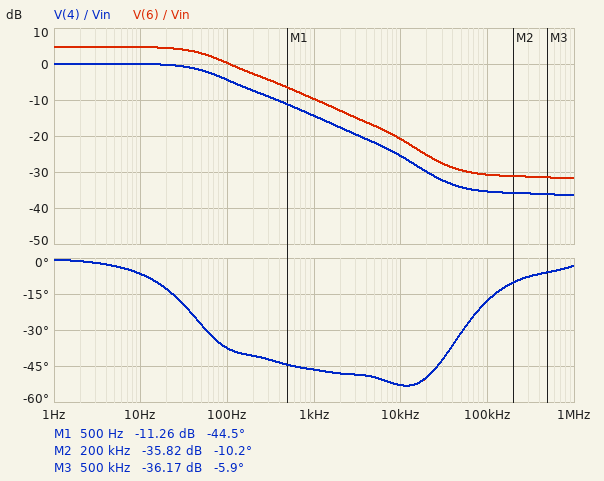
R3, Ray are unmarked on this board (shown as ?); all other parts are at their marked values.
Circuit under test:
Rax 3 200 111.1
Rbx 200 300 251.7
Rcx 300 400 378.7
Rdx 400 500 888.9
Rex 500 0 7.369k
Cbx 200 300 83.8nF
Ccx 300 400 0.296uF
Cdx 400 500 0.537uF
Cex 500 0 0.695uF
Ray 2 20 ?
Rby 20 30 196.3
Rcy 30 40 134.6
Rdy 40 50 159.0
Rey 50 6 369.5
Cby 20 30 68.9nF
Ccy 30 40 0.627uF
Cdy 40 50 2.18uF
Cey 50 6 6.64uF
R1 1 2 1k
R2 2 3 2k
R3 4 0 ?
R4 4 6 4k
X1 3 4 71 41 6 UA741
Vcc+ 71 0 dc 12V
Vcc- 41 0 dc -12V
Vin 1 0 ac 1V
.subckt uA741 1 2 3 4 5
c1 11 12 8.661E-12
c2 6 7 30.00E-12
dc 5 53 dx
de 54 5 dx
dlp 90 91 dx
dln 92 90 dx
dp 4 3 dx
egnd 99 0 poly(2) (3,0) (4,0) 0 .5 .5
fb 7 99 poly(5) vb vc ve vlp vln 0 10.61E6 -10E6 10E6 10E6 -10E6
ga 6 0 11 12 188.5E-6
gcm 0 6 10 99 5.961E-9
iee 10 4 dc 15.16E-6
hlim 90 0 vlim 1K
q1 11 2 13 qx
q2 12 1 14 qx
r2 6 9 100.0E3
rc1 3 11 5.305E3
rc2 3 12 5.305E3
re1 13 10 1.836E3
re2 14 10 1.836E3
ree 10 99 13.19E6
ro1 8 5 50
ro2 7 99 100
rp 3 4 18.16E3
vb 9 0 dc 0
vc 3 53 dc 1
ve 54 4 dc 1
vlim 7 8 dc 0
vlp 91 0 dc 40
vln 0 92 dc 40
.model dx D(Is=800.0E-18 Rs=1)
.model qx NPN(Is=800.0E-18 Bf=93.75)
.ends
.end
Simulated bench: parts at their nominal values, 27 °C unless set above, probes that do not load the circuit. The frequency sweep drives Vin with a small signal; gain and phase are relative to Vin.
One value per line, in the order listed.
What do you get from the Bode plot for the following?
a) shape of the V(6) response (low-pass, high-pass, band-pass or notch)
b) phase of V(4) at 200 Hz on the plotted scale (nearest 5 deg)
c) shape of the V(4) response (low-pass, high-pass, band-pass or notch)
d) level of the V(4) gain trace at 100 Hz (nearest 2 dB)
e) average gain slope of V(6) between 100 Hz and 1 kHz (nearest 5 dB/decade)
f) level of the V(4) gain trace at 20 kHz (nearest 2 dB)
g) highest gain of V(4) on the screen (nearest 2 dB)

low-pass
-40 deg
low-pass
-4 dB
-10 dB/decade
-30 dB
0 dB
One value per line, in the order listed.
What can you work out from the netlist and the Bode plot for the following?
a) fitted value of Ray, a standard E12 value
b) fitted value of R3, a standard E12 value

560 Ω
5.6 kΩ
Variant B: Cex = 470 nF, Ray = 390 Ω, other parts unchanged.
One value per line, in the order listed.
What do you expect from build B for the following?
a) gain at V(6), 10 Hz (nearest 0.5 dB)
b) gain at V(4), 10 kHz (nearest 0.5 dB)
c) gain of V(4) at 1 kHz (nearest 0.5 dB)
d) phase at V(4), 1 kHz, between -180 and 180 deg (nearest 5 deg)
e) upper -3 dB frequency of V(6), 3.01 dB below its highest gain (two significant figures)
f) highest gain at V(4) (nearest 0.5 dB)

5.0 dB
-26.5 dB
-14.0 dB
-55 deg
100 Hz
0.5 dB
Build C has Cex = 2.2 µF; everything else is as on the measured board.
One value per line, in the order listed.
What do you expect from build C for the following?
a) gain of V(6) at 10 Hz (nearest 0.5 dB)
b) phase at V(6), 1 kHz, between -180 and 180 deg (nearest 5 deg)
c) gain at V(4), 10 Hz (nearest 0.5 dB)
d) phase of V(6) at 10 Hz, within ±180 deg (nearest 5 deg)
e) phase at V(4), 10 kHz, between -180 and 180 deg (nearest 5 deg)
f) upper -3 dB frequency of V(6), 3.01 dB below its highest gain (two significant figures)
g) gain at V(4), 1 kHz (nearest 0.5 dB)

3.5 dB
-40 deg
-1.0 dB
-20 deg
-50 deg
20 Hz
-15.5 dB
